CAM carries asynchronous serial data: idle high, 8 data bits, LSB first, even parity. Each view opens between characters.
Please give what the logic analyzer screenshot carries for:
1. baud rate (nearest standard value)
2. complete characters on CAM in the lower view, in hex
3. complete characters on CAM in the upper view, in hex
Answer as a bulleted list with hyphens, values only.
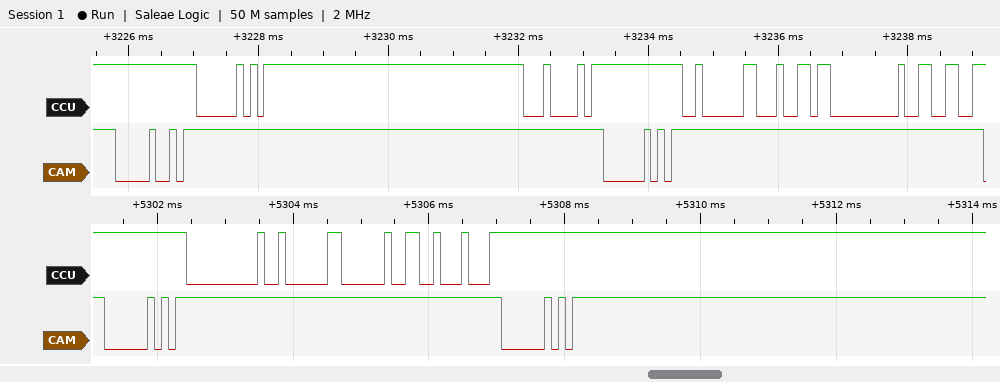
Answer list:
- 9600 baud
- A0, A0
- 90, A0
